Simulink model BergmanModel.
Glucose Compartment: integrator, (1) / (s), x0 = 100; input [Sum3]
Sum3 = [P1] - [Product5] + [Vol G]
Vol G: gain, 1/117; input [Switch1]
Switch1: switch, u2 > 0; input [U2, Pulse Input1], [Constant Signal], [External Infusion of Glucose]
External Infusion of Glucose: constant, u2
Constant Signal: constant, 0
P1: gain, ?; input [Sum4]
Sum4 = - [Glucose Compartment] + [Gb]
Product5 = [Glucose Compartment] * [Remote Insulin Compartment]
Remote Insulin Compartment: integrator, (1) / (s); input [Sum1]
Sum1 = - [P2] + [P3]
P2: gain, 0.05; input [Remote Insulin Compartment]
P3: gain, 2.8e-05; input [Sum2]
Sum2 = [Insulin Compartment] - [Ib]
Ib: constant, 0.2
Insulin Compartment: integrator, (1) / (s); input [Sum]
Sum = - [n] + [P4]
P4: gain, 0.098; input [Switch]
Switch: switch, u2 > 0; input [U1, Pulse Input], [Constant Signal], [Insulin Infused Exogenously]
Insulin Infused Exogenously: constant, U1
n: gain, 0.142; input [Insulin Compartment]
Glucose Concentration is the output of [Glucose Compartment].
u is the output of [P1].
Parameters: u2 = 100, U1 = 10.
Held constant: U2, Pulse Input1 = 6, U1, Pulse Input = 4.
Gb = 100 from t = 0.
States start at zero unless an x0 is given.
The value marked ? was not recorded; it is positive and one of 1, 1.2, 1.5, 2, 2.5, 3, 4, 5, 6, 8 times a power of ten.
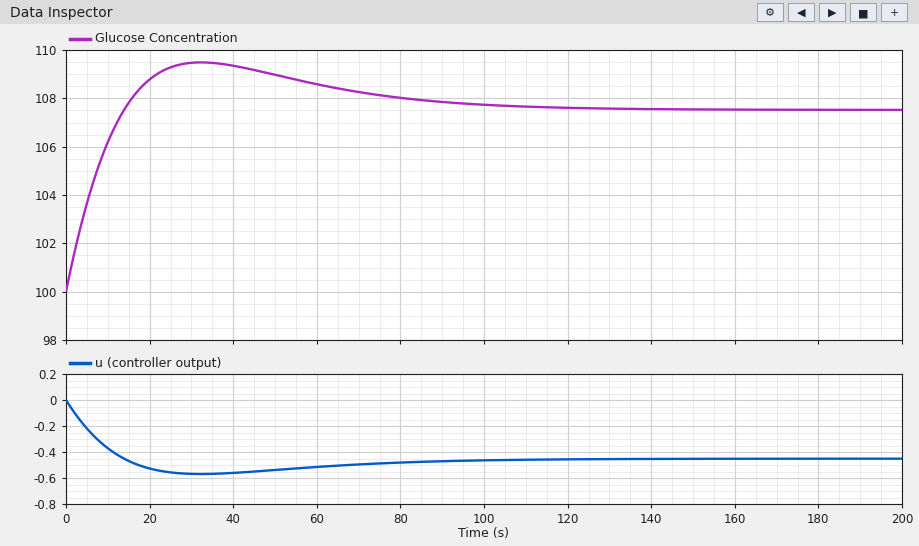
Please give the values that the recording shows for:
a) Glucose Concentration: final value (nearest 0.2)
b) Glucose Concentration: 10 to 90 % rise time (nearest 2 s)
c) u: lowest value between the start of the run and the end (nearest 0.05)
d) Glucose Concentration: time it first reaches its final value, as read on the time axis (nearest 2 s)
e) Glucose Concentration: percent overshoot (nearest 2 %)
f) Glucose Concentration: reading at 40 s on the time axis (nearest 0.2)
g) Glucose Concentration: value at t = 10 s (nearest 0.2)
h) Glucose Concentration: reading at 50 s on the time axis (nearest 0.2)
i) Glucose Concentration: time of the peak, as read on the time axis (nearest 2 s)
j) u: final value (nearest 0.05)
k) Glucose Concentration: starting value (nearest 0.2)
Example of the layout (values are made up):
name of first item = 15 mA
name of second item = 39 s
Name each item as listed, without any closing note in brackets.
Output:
Glucose Concentration: final value = 107.6
Glucose Concentration: 10 to 90 % rise time = 10 s
u: lowest value between the start of the run and the end = -0.55
Glucose Concentration: time it first reaches its final value, as read on the time axis = 14 s
Glucose Concentration: percent overshoot = 26 %
Glucose Concentration: reading at 40 s on the time axis = 109.4
Glucose Concentration: value at t = 10 s = 106.2
Glucose Concentration: reading at 50 s on the time axis = 109.0
Glucose Concentration: time of the peak, as read on the time axis = 32 s
u: final value = -0.45
Glucose Concentration: starting value = 100.0
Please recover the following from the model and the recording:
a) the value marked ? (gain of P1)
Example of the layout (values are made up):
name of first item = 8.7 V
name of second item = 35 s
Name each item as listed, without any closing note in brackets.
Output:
the value marked ? = 0.06
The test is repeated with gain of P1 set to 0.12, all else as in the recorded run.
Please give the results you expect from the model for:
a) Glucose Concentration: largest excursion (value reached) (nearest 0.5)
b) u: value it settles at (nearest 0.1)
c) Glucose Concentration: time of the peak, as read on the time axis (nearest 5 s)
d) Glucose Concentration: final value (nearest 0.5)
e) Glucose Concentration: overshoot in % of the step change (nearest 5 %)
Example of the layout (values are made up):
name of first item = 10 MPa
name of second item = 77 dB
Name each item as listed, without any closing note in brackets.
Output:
Glucose Concentration: largest excursion (value reached) = 105.5
u: value it settles at = -0.5
Glucose Concentration: time of the peak, as read on the time axis = 20 s
Glucose Concentration: final value = 104.0
Glucose Concentration: overshoot in % of the step change = 45 %
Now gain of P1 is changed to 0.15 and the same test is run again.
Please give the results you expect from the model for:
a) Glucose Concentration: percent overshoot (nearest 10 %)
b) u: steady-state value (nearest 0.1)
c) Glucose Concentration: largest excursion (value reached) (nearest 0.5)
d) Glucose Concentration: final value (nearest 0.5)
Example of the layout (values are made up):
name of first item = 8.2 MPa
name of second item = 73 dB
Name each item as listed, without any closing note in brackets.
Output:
Glucose Concentration: percent overshoot = 50 %
u: steady-state value = -0.5
Glucose Concentration: largest excursion (value reached) = 104.5
Glucose Concentration: final value = 103.0
